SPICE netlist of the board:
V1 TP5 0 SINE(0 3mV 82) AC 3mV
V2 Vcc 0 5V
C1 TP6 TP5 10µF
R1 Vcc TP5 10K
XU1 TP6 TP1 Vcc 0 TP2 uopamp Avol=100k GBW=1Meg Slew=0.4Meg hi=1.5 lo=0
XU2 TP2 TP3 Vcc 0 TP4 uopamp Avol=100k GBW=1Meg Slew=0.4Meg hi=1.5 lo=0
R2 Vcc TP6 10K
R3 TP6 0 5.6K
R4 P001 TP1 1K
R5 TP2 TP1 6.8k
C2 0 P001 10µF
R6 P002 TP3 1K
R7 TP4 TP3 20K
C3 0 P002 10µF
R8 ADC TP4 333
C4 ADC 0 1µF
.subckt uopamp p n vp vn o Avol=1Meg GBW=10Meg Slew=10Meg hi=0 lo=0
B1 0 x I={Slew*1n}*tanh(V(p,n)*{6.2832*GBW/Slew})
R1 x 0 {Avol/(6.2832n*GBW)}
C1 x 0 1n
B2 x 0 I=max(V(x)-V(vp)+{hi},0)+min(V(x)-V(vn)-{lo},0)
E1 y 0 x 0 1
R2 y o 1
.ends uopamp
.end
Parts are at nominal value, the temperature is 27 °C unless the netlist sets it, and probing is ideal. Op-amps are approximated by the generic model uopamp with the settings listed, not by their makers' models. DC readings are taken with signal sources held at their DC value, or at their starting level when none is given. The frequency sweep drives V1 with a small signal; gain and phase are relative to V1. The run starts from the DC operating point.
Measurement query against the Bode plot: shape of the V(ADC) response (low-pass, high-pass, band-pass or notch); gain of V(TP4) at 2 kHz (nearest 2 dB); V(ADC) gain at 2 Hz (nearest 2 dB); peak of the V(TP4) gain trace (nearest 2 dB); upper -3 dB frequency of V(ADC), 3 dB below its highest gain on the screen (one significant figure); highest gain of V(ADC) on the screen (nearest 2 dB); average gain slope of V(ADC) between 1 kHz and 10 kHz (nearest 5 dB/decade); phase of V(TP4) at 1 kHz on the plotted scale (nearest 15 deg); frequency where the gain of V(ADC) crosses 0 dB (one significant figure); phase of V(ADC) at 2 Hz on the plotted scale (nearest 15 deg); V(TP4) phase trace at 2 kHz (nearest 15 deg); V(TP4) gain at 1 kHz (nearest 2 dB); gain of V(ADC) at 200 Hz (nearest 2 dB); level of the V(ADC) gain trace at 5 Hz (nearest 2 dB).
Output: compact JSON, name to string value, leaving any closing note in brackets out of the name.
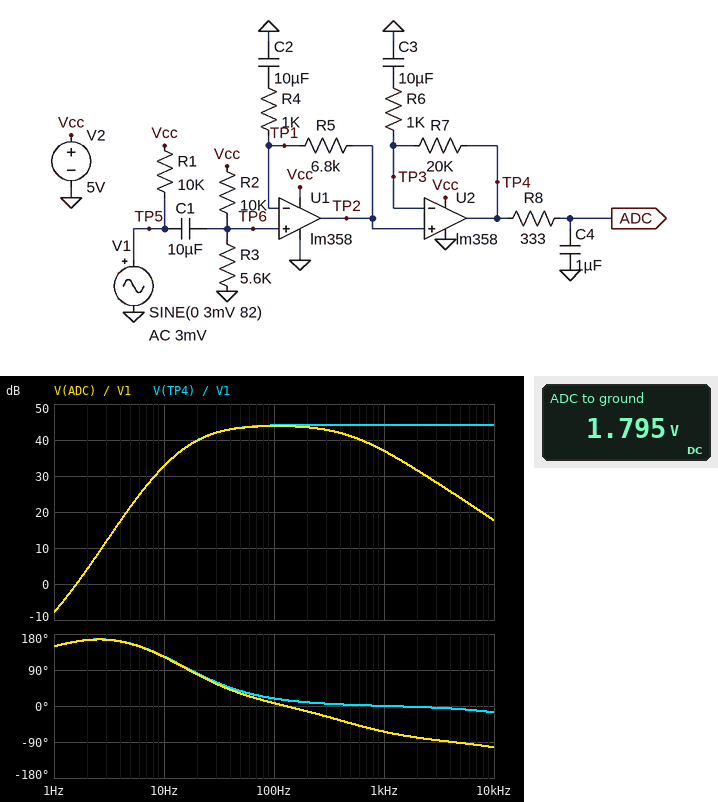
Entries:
{"shape of the V(ADC) response": "band-pass", "gain of V(TP4) at 2 kHz": "44 dB", "V(ADC) gain at 2 Hz": "4 dB", "peak of the V(TP4) gain trace": "44 dB", "upper -3 dB frequency of V(ADC), 3 dB below its highest gain on the screen": "500 Hz", "highest gain of V(ADC) on the screen": "44 dB", "average gain slope of V(ADC) between 1 kHz and 10 kHz": "-20 dB/decade", "phase of V(TP4) at 1 kHz on the plotted scale": "0 deg", "frequency where the gain of V(ADC) crosses 0 dB": "2 Hz", "phase of V(ADC) at 2 Hz on the plotted scale": "165 deg", "V(TP4) phase trace at 2 kHz": "0 deg", "V(TP4) gain at 1 kHz": "44 dB", "gain of V(ADC) at 200 Hz": "44 dB", "level of the V(ADC) gain trace at 5 Hz": "22 dB"}
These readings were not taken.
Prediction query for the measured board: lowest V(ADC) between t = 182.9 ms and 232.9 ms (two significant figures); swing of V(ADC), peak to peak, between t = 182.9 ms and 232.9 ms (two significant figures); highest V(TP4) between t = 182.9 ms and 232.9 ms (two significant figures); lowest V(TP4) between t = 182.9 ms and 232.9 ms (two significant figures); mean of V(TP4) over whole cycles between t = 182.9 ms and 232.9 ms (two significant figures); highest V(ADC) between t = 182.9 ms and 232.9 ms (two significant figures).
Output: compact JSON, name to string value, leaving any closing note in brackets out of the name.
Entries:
{"lowest V(ADC) between t = 182.9 ms and 232.9 ms": "1.3 V", "swing of V(ADC), peak to peak, between t = 182.9 ms and 232.9 ms": "930 mV", "highest V(TP4) between t = 182.9 ms and 232.9 ms": "2.3 V", "lowest V(TP4) between t = 182.9 ms and 232.9 ms": "1.3 V", "mean of V(TP4) over whole cycles between t = 182.9 ms and 232.9 ms": "1.8 V", "highest V(ADC) between t = 182.9 ms and 232.9 ms": "2.3 V"}
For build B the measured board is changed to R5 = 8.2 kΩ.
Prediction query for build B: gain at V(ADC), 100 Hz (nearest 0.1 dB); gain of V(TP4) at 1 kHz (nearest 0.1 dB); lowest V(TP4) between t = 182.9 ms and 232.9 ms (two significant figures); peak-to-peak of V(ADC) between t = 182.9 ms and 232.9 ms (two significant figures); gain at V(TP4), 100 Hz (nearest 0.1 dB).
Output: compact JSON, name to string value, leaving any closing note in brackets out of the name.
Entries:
{"gain at V(ADC), 100 Hz": "45.3 dB", "gain of V(TP4) at 1 kHz": "45.7 dB", "lowest V(TP4) between t = 182.9 ms and 232.9 ms": "1.2 V", "peak-to-peak of V(ADC) between t = 182.9 ms and 232.9 ms": "1.1 V", "gain at V(TP4), 100 Hz": "45.5 dB"}
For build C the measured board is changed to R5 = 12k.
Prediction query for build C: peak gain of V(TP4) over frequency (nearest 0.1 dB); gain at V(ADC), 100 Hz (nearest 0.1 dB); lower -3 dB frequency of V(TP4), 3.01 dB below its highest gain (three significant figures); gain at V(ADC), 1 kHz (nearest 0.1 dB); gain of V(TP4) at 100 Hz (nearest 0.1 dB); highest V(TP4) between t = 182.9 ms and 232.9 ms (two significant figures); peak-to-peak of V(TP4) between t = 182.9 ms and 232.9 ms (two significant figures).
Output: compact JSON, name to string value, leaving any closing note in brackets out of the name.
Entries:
{"peak gain of V(TP4) over frequency": "48.7 dB", "gain at V(ADC), 100 Hz": "48.3 dB", "lower -3 dB frequency of V(TP4), 3.01 dB below its highest gain": "25.3 Hz", "gain at V(ADC), 1 kHz": "41.4 dB", "gain of V(TP4) at 100 Hz": "48.5 dB", "highest V(TP4) between t = 182.9 ms and 232.9 ms": "2.6 V", "peak-to-peak of V(TP4) between t = 182.9 ms and 232.9 ms": "1.6 V"}
